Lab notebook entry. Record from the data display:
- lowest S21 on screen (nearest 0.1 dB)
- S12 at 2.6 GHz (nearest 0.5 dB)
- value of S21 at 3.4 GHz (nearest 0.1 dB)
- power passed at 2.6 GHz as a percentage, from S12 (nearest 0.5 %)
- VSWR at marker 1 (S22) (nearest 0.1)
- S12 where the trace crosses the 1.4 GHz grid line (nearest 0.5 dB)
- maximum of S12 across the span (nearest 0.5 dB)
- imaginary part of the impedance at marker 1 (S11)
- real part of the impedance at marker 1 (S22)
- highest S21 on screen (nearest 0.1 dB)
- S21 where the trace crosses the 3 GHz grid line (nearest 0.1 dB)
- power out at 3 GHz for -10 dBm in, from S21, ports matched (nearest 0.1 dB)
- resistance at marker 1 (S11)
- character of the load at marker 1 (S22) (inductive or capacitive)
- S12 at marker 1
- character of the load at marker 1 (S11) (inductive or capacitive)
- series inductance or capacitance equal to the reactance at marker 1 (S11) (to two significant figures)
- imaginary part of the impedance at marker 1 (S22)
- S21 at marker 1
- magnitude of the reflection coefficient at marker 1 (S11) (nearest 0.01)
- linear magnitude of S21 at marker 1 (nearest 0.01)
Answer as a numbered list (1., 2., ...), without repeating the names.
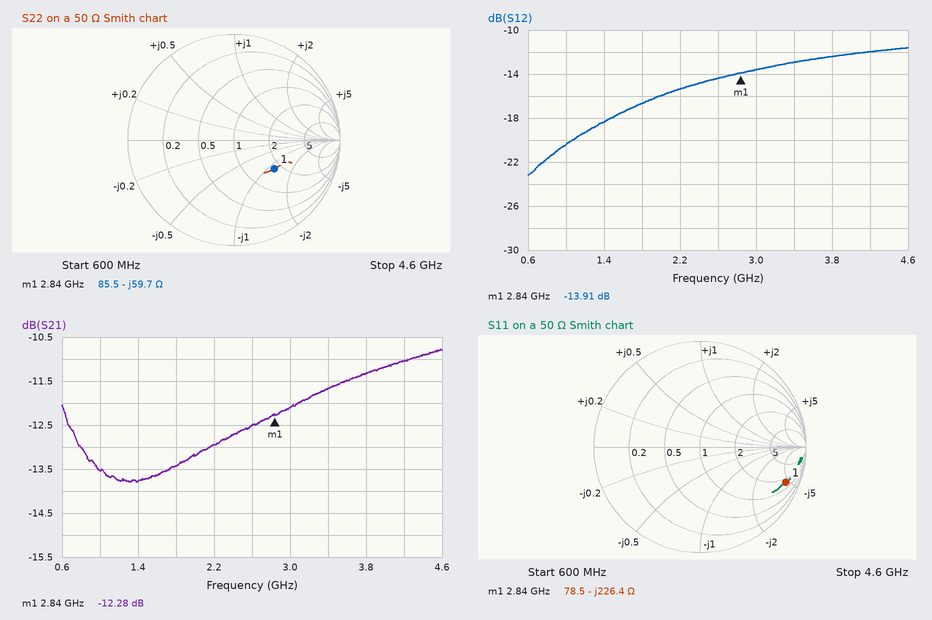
1. -13.8 dB
2. -14.5 dB
3. -11.7 dB
4. 3.5 %
5. 2.8
6. -18.5 dB
7. -11.5 dB
8. -226.4 Ω
9. 85.5 Ω
10. -10.8 dB
11. -12.1 dB
12. -22.1 dBm
13. 78.5 Ω
14. capacitive
15. -13.91 dB
16. capacitive
17. 250 fF
18. -59.7 Ω
19. -12.28 dB
20. 0.88
21. 0.24
